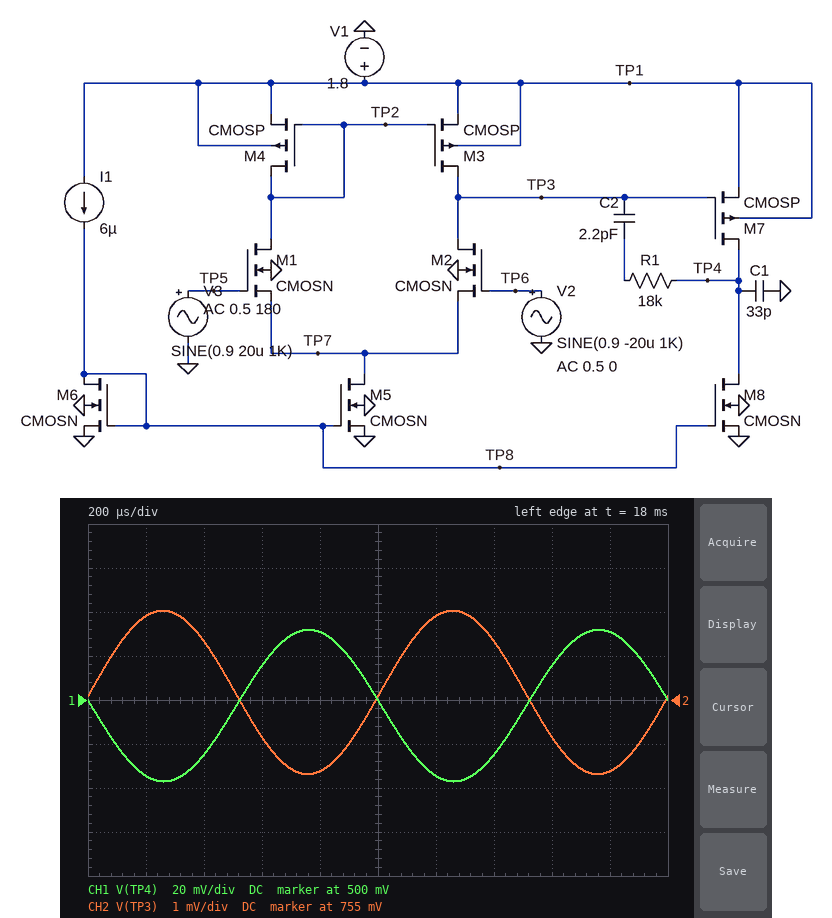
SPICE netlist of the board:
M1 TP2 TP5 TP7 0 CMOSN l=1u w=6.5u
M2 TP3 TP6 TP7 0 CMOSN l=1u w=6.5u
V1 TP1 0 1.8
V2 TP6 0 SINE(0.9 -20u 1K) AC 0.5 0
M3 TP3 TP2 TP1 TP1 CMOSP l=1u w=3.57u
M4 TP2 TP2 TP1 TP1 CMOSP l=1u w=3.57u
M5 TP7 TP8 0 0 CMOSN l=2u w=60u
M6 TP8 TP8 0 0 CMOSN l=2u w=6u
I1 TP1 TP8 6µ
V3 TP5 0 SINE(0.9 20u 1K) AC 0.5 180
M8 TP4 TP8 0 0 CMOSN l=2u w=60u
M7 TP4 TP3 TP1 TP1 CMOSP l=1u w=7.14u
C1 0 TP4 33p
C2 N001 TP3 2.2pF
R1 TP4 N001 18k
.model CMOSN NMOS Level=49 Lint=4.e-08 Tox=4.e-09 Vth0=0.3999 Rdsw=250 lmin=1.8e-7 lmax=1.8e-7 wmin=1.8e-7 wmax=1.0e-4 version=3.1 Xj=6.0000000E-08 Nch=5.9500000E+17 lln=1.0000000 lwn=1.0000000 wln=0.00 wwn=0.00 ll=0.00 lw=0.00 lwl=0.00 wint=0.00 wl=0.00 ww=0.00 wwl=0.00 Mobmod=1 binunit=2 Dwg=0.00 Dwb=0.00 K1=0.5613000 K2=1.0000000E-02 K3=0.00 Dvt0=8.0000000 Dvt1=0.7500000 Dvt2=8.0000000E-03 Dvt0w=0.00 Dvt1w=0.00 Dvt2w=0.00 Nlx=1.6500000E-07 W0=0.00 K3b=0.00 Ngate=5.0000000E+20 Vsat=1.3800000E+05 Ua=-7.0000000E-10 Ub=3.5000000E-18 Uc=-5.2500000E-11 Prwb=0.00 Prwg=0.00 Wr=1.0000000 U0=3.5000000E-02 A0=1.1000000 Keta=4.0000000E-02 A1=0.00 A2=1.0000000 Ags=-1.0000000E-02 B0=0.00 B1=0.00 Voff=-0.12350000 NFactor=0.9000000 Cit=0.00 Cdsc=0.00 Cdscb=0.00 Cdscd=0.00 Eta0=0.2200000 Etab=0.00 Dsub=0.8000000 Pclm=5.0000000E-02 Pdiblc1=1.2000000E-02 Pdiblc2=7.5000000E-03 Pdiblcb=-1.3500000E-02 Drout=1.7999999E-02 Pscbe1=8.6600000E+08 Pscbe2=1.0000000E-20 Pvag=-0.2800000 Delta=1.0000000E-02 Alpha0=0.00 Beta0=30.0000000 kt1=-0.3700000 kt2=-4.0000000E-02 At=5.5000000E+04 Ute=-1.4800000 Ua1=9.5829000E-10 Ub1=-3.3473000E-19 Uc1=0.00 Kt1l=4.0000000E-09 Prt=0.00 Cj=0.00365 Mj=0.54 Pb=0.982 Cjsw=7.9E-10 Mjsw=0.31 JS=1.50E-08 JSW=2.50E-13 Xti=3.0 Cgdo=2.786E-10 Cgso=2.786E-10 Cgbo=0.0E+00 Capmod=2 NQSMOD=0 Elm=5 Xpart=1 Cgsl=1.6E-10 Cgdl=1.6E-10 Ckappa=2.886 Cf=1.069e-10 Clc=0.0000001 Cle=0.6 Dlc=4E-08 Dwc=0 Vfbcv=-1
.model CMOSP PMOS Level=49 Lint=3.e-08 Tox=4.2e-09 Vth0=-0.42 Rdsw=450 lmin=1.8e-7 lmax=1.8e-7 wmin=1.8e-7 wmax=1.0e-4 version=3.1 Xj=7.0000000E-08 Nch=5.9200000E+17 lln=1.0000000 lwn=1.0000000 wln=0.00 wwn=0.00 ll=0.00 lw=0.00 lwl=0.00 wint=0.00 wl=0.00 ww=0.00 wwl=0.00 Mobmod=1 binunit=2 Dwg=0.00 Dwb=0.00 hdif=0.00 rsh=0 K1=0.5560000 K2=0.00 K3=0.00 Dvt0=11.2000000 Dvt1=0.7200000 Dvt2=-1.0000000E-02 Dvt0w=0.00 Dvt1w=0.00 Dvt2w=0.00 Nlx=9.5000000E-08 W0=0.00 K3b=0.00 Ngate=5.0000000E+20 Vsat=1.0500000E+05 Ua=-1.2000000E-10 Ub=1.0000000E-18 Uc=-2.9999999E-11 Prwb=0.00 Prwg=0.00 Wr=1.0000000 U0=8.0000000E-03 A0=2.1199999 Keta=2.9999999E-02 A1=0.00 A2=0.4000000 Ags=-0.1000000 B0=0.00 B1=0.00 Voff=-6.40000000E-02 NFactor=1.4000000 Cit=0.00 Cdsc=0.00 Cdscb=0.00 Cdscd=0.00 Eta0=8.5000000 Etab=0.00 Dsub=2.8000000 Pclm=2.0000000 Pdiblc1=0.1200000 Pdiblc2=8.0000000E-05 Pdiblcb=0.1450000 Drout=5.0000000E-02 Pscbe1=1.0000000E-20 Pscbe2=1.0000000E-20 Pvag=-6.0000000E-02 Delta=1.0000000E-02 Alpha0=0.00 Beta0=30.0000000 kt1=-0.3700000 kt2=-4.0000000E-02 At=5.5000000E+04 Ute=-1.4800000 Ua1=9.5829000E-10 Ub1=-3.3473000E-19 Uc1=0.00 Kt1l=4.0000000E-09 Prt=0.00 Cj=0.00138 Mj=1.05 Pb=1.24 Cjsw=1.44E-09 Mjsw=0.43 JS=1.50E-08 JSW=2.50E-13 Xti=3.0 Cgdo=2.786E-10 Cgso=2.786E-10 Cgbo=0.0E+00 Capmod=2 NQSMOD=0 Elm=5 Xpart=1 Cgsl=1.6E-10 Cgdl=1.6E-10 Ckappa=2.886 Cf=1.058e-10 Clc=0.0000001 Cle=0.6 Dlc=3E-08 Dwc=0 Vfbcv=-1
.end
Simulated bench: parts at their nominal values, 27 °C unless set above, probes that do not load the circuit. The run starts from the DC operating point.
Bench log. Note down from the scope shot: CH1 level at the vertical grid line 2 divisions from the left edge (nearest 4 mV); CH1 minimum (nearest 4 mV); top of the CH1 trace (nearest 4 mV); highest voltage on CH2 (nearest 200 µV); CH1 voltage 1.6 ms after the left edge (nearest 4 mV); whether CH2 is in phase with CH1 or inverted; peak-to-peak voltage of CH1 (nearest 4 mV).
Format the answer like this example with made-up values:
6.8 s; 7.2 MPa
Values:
476 mV; 464 mV; 532 mV; 757.0 mV; 516 mV; inverted; 68 mV
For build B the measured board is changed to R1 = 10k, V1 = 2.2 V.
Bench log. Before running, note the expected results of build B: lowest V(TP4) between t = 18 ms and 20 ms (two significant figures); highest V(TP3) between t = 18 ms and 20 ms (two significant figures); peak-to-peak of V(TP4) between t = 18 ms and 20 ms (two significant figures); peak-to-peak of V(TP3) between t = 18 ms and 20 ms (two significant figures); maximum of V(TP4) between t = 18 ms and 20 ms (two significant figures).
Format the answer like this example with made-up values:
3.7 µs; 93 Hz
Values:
700 mV; 1.2 V; 74 mV; 3.9 mV; 770 mV
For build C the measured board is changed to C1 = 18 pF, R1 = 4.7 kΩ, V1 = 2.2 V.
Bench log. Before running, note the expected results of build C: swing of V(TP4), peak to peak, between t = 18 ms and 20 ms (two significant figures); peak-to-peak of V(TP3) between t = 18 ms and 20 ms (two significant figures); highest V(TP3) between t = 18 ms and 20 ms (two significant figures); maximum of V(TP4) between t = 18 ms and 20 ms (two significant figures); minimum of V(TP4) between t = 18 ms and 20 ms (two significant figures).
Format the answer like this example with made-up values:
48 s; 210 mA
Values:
74 mV; 3.9 mV; 1.2 V; 770 mV; 700 mV
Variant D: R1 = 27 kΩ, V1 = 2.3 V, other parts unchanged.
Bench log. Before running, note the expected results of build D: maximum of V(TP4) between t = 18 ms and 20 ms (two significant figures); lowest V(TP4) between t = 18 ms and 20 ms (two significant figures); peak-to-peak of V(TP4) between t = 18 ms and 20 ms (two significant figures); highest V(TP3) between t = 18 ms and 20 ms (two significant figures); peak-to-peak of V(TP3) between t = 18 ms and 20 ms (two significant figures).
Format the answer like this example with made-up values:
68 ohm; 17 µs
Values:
830 mV; 760 mV; 75 mV; 1.3 V; 3.9 mV
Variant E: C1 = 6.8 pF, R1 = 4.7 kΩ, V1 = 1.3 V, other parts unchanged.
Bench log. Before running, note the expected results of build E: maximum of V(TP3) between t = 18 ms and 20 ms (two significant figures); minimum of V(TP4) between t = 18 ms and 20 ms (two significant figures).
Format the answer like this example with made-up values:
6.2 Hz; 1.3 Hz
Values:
260 mV; 190 mV
